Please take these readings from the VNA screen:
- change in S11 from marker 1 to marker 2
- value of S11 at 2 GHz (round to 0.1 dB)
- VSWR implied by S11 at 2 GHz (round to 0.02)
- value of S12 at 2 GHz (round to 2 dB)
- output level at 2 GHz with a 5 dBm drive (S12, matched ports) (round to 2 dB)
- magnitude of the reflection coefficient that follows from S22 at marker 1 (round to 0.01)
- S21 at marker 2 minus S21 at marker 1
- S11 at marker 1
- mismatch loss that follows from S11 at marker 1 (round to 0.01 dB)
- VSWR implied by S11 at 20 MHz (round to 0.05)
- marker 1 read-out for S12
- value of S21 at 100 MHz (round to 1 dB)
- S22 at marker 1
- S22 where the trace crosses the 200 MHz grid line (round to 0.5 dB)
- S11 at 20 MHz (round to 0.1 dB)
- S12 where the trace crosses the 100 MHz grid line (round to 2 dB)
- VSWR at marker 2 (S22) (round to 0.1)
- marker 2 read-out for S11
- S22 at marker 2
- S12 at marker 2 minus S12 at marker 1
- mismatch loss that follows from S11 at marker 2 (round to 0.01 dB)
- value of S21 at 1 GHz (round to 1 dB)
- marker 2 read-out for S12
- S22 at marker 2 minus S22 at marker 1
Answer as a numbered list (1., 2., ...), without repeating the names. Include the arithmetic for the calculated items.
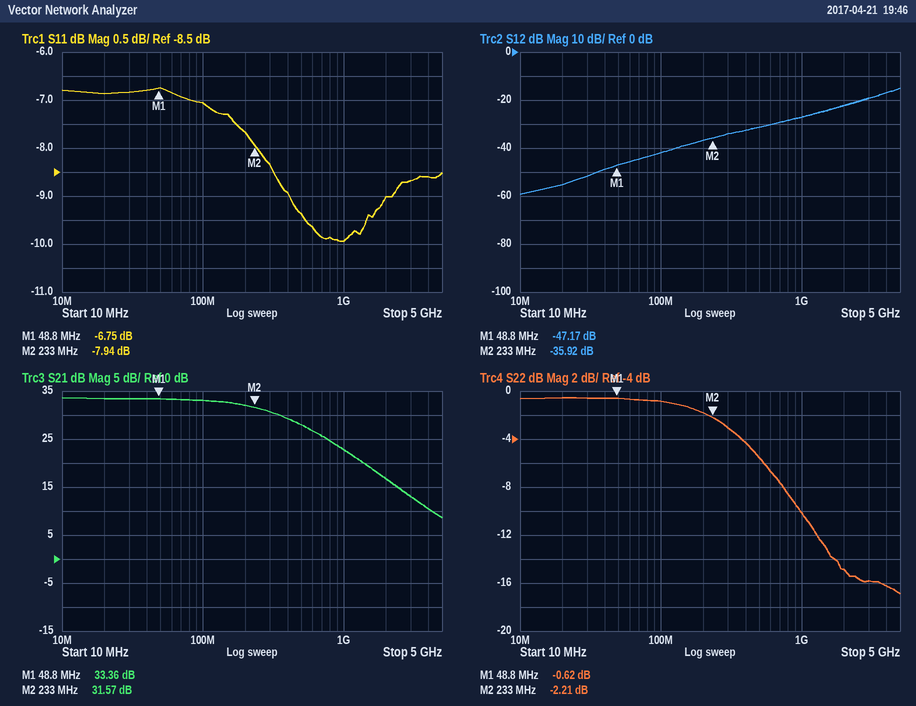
1. -7.94 − (-6.75) = -1.19 dB
2. -9.0 dB
3. |Γ| = 10^(-9/20) = 0.3548; VSWR = (1 + 0.3548)/(1 − 0.3548) ≈ 2.10
4. -22 dB
5. 5 dBm + (-22 dB) = -18 dBm
6. 10^(-0.62/20) ≈ 0.93
7. 31.57 − (33.36) = -1.79 dB
8. -6.75 dB
9. −10 log10(1 − 10^(-6.75/10)) ≈ 1.03 dB
10. |Γ| = 10^(-6.9/20) = 0.4519; VSWR = (1 + 0.4519)/(1 − 0.4519) ≈ 2.65
11. -47.17 dB
12. 33 dB
13. -0.62 dB
14. -2.0 dB
15. -6.9 dB
16. -42 dB
17. (1 + 0.7754)/(1 − 0.7754) ≈ 7.9
18. -7.94 dB
19. -2.21 dB
20. -35.92 − (-47.17) = 11.25 dB
21. −10 log10(1 − 10^(-7.94/10)) ≈ 0.76 dB
22. 23 dB
23. -35.92 dB
24. -2.21 − (-0.62) = -1.59 dB
